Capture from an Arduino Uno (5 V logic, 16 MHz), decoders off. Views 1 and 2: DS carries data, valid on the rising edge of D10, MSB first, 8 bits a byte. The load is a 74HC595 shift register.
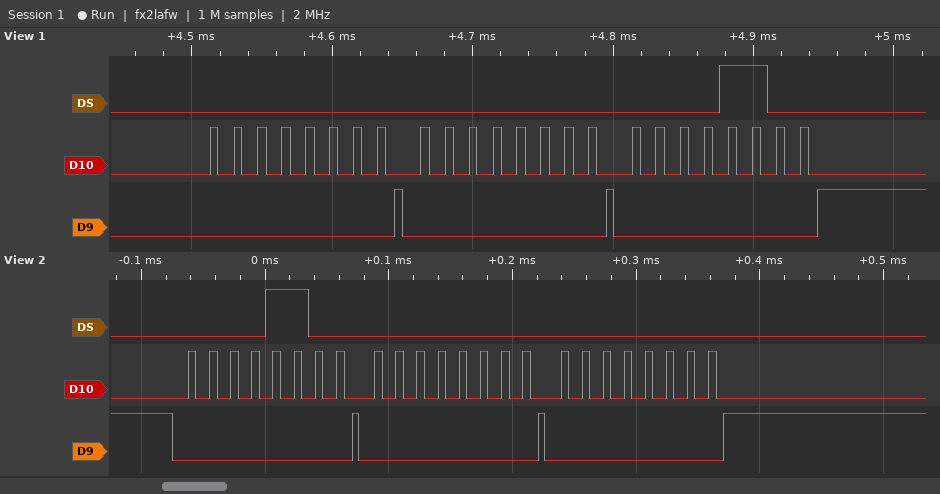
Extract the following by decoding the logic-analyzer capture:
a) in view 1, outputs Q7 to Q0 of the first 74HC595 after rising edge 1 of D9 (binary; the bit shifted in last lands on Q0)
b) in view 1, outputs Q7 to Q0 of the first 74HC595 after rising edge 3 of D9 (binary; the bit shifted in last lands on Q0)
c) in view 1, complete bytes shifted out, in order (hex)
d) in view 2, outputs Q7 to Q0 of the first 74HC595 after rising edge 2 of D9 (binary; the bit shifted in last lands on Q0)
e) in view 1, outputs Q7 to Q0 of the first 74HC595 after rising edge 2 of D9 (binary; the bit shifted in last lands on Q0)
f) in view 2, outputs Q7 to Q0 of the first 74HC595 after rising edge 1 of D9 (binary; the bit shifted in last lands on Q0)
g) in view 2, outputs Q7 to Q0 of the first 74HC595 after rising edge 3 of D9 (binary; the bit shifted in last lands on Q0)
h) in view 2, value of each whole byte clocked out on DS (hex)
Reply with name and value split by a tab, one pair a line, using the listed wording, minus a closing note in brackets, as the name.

in view 1, outputs Q7 to Q0 of the first 74HC595 after rising edge 1 of D9	00000000
in view 1, outputs Q7 to Q0 of the first 74HC595 after rising edge 3 of D9	00001100
in view 1, complete bytes shifted out, in order	00 00 0C
in view 2, outputs Q7 to Q0 of the first 74HC595 after rising edge 2 of D9	00000000
in view 1, outputs Q7 to Q0 of the first 74HC595 after rising edge 2 of D9	00000000
in view 2, outputs Q7 to Q0 of the first 74HC595 after rising edge 1 of D9	00001100
in view 2, outputs Q7 to Q0 of the first 74HC595 after rising edge 3 of D9	00000000
in view 2, value of each whole byte clocked out on DS	0x0C 0x00 0x00
